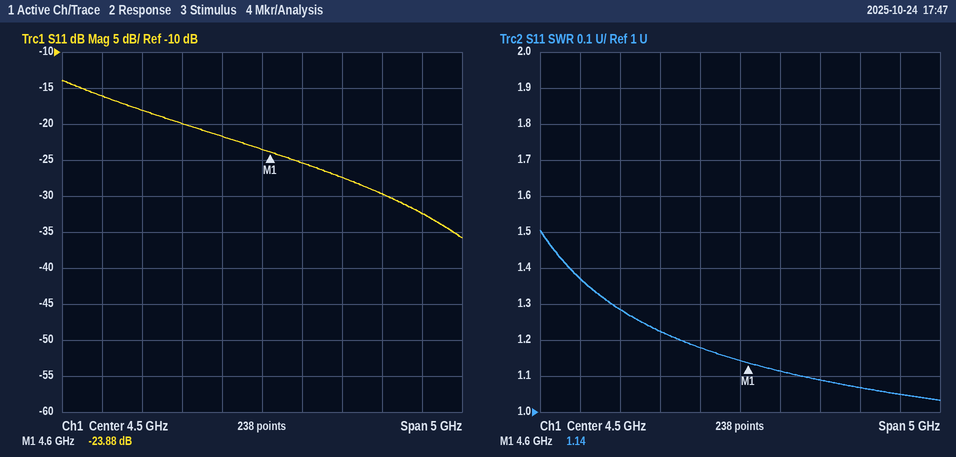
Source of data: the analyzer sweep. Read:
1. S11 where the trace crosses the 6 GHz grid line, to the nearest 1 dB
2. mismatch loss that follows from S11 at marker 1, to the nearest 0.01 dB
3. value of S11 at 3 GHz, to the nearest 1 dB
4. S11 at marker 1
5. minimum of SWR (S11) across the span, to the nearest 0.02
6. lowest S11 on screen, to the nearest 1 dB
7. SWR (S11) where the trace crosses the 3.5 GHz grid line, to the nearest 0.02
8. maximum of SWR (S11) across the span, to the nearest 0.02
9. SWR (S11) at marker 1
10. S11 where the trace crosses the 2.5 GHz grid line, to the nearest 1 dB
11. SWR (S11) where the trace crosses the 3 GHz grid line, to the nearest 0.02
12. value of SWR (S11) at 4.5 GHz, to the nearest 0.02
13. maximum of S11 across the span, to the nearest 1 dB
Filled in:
-30 dB
0.02 dB
-18 dB
-23.88 dB
1.04
-36 dB
1.22
1.50
1.14
-16 dB
1.28
1.14
-14 dB
